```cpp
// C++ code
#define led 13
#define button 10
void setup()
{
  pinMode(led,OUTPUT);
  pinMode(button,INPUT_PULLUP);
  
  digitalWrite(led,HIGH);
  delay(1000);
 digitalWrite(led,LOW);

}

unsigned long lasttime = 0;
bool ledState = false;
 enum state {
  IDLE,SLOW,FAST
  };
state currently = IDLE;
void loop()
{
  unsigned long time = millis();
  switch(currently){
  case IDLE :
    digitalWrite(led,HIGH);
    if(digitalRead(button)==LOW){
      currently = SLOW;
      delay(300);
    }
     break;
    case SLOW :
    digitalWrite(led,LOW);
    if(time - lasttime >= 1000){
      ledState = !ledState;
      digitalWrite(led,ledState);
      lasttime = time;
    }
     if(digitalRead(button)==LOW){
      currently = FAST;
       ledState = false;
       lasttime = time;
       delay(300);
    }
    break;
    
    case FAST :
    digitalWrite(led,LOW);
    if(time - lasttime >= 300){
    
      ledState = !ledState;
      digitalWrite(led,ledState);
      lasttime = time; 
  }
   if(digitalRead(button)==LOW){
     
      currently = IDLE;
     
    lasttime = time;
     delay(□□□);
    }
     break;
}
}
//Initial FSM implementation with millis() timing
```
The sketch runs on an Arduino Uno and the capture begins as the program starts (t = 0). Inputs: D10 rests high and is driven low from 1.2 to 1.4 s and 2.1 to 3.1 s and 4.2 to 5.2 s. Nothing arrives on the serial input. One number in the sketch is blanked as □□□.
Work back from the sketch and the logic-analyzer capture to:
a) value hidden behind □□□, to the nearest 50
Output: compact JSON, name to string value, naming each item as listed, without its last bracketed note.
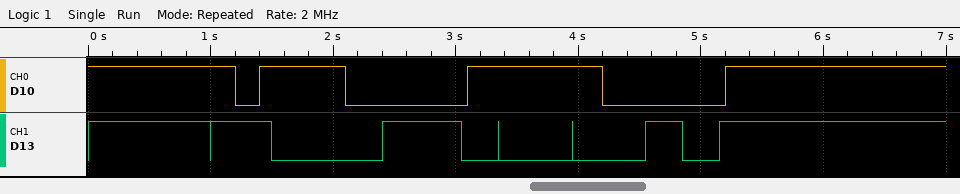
{"value hidden behind □□□, to the nearest 50": "350"}
